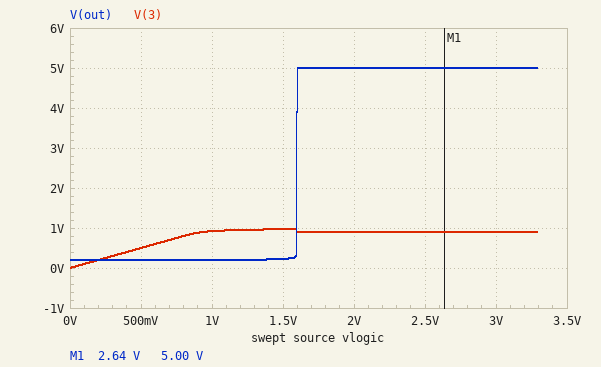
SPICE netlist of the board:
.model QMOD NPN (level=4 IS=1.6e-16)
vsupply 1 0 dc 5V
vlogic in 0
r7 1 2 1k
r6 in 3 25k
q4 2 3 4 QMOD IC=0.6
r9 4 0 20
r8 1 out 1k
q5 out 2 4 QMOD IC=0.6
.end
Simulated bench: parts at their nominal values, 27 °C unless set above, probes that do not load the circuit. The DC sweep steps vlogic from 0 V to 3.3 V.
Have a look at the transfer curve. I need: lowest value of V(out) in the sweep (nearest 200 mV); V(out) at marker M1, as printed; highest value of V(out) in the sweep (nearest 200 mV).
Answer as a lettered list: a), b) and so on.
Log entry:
a) 200 mV
b) 5.00 V
c) 5.0 V
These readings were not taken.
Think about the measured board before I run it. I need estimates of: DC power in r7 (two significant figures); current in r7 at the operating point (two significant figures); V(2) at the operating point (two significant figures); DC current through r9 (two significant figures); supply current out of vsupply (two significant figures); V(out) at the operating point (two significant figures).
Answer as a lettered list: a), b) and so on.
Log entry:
a) 16 mW
b) 4.0 mA
c) 1.0 V
d) 8.8 mA
e) 8.8 mA
f) 200 mV
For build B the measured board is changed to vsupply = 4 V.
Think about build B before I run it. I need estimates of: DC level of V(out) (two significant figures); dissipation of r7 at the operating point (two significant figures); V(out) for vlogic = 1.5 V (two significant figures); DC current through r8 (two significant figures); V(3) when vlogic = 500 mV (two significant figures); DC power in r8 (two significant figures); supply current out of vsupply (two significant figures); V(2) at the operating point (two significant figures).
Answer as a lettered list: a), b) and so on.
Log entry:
a) 160 mV
b) 9.2 mW
c) 4.0 V
d) 3.8 mA
e) 500 mV
f) 15 mW
g) 6.9 mA
h) 960 mV
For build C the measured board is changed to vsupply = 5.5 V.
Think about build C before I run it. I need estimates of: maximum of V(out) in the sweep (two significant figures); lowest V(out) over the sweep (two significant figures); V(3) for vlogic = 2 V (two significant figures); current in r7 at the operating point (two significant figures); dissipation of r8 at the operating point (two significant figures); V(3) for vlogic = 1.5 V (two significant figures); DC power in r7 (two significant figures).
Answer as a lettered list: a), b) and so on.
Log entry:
a) 5.5 V
b) 220 mV
c) 910 mV
d) 4.5 mA
e) 28 mW
f) 990 mV
g) 20 mW
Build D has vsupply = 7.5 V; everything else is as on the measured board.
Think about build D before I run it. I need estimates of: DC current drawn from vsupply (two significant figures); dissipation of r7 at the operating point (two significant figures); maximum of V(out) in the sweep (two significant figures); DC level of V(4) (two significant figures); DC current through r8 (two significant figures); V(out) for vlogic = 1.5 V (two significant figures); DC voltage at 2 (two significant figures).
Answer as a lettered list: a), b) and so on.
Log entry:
a) 14 mA
b) 41 mW
c) 7.5 V
d) 270 mV
e) 7.2 mA
f) 300 mV
g) 1.1 V
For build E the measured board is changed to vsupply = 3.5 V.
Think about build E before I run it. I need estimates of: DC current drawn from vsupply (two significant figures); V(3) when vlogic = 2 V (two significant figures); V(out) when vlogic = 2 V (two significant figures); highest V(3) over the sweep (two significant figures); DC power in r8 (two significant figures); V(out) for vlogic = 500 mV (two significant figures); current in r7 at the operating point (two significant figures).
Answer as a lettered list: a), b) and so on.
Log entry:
a) 5.9 mA
b) 860 mV
c) 3.5 V
d) 900 mV
e) 11 mW
f) 140 mV
g) 2.6 mA
